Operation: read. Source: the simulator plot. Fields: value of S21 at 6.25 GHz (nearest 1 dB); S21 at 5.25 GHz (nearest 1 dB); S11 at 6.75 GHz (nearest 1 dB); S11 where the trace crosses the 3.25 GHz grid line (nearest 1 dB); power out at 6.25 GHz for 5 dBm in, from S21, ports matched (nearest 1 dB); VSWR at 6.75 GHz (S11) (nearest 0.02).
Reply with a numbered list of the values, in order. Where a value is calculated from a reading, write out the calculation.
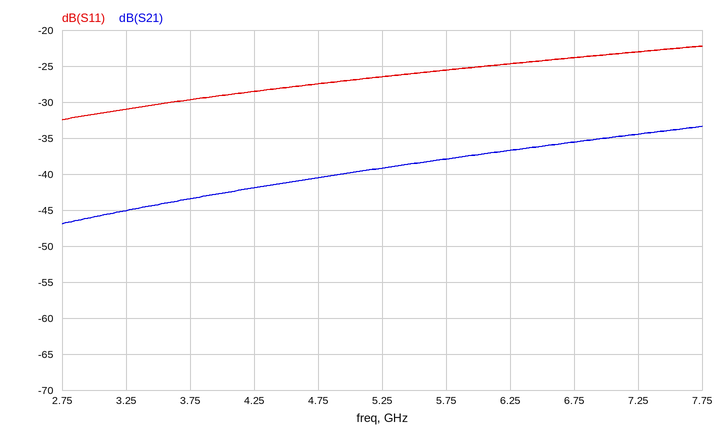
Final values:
1. -37 dB
2. -39 dB
3. -24 dB
4. -31 dB
5. 5 dBm + (-37 dB) = -32 dBm
6. |Γ| = 10^(-24/20) = 0.0631; VSWR = (1 + 0.0631)/(1 − 0.0631) ≈ 1.13, so 1.14 to the nearest 0.02
